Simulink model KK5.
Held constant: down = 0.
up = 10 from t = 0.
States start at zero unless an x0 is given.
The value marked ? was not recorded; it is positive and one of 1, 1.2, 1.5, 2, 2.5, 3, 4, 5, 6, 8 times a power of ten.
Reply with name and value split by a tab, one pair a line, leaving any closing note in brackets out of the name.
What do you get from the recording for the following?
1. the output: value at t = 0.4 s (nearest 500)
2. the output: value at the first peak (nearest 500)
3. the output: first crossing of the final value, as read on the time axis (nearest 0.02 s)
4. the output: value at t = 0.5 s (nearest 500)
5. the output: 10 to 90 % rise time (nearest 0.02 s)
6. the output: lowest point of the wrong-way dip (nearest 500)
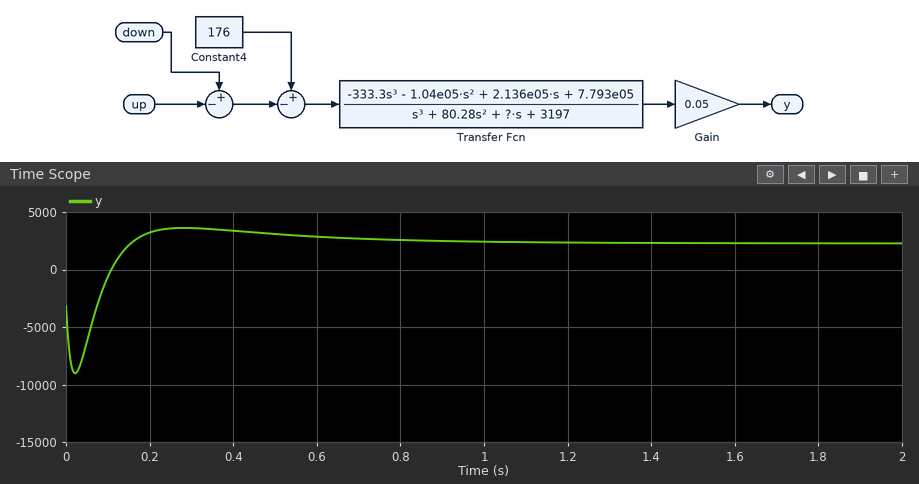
the output: value at t = 0.4 s	3500
the output: value at the first peak	3500
the output: first crossing of the final value, as read on the time axis	0.16 s
the output: value at t = 0.5 s	3000
the output: 10 to 90 % rise time	0.06 s
the output: lowest point of the wrong-way dip	-9000
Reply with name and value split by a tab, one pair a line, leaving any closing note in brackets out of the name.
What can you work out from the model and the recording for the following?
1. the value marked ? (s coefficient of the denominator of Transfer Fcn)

the value marked ?	1200
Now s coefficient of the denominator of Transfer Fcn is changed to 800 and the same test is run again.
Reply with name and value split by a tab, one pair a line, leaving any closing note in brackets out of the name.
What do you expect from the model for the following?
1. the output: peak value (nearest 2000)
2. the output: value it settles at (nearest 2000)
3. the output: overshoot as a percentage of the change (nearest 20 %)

the output: peak value	6000
the output: value it settles at	2000
the output: overshoot as a percentage of the change	60 %
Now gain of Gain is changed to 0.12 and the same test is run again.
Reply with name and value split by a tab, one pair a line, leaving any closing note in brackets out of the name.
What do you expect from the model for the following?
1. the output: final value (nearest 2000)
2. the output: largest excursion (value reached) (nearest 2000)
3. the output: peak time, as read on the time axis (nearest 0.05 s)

the output: final value	6000
the output: largest excursion (value reached)	8000
the output: peak time, as read on the time axis	0.30 s
